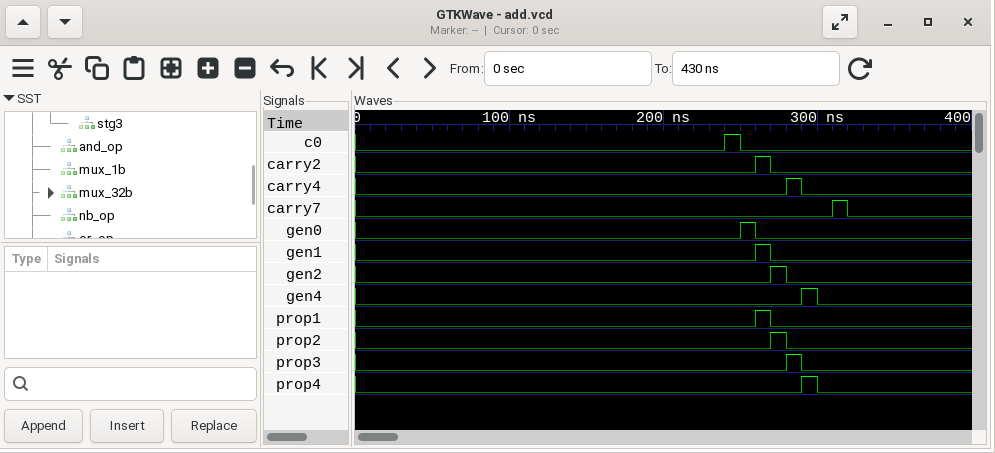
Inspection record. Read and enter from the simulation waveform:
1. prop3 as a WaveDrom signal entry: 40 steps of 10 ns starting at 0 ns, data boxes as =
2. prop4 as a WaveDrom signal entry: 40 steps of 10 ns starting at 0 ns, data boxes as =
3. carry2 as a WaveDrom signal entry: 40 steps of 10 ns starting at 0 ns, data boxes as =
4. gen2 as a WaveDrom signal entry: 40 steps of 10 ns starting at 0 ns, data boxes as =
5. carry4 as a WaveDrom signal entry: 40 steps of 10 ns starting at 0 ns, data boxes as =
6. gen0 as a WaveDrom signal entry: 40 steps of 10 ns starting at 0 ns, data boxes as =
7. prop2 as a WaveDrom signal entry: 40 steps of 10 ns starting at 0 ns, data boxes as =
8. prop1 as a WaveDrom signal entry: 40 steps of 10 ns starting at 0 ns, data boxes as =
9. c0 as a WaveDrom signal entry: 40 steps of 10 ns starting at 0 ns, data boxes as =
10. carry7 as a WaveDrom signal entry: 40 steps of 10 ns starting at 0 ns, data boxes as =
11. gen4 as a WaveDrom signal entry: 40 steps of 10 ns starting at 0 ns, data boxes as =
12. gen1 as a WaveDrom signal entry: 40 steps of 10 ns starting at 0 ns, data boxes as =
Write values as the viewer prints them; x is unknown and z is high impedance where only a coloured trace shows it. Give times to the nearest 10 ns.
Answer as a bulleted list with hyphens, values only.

- {name: 'prop3', wave: '0...........................10..........'}
- {name: 'prop4', wave: '0............................10.........'}
- {name: 'carry2', wave: '0.........................10............'}
- {name: 'gen2', wave: '0..........................10...........'}
- {name: 'carry4', wave: '0...........................10..........'}
- {name: 'gen0', wave: '0........................10.............'}
- {name: 'prop2', wave: '0..........................10...........'}
- {name: 'prop1', wave: '0.........................10............'}
- {name: 'c0', wave: '0.......................10..............'}
- {name: 'carry7', wave: '0..............................10.......'}
- {name: 'gen4', wave: '0............................10.........'}
- {name: 'gen1', wave: '0.........................10............'}
